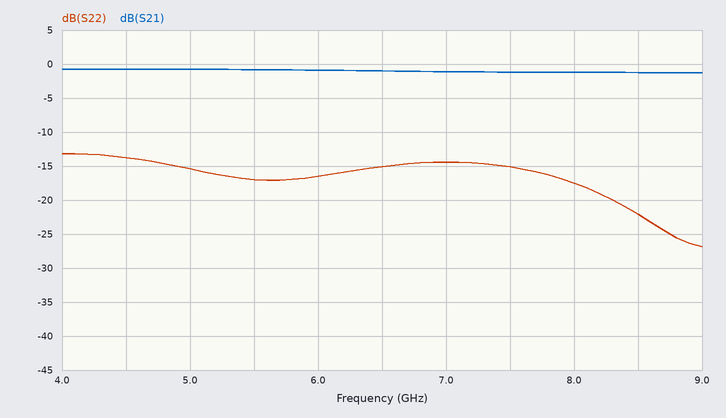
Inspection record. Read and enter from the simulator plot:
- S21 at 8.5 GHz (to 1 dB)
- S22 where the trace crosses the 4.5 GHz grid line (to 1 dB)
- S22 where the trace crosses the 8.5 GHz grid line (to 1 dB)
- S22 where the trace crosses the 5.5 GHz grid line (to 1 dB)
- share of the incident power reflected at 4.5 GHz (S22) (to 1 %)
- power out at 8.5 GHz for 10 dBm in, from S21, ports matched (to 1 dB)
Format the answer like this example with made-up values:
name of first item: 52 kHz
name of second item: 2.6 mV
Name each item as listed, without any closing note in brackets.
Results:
S21 at 8.5 GHz: -1 dB
S22 where the trace crosses the 4.5 GHz grid line: -14 dB
S22 where the trace crosses the 8.5 GHz grid line: -22 dB
S22 where the trace crosses the 5.5 GHz grid line: -17 dB
share of the incident power reflected at 4.5 GHz (S22): 4 %
power out at 8.5 GHz for 10 dBm in, from S21, ports matched: 9 dBm
